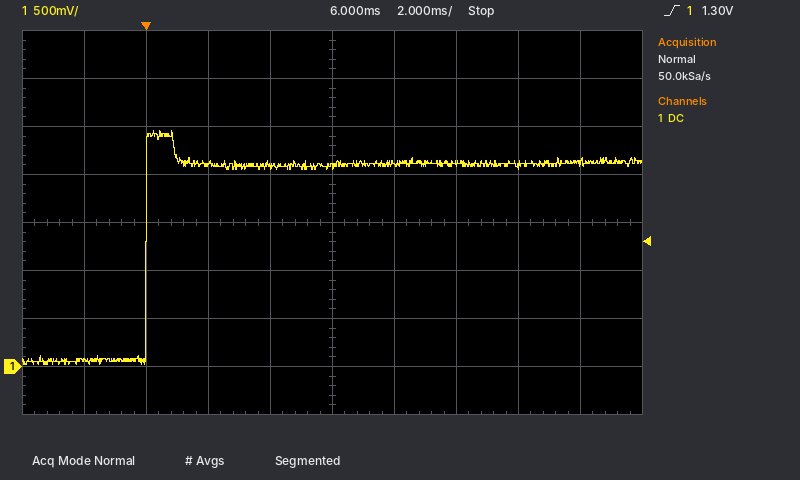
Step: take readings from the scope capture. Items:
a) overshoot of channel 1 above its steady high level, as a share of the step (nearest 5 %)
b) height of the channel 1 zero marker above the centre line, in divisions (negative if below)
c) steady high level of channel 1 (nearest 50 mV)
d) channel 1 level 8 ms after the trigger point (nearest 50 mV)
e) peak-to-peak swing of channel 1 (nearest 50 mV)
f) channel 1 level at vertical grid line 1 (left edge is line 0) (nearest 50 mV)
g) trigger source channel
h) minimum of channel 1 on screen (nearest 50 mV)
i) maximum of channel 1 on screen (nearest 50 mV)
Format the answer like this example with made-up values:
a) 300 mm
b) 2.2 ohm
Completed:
a) 15 %
b) -3.0 div
c) 2.10 V
d) 2.10 V
e) 2.45 V
f) 50 mV
g) channel 1
h) 0 mV
i) 2.45 V
